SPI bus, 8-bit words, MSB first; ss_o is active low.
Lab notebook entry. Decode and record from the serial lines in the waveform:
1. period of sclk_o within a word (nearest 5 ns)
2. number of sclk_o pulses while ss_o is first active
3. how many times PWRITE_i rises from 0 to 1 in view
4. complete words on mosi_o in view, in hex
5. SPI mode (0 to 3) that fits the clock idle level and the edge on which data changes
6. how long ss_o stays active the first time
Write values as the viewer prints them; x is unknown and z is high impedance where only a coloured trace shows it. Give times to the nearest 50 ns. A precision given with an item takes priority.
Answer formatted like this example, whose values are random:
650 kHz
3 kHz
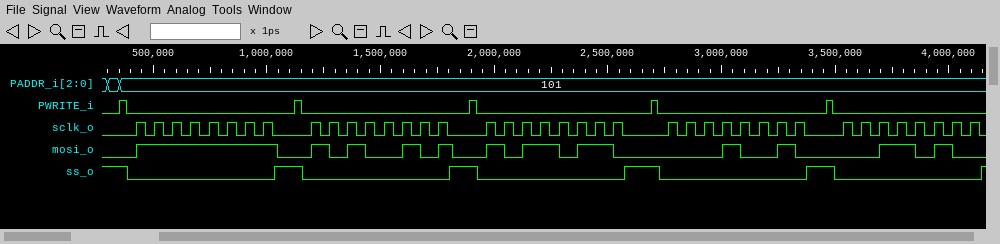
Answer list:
80 ns
8
5
FF, A5, B6, 12, 34
1
650 ns
